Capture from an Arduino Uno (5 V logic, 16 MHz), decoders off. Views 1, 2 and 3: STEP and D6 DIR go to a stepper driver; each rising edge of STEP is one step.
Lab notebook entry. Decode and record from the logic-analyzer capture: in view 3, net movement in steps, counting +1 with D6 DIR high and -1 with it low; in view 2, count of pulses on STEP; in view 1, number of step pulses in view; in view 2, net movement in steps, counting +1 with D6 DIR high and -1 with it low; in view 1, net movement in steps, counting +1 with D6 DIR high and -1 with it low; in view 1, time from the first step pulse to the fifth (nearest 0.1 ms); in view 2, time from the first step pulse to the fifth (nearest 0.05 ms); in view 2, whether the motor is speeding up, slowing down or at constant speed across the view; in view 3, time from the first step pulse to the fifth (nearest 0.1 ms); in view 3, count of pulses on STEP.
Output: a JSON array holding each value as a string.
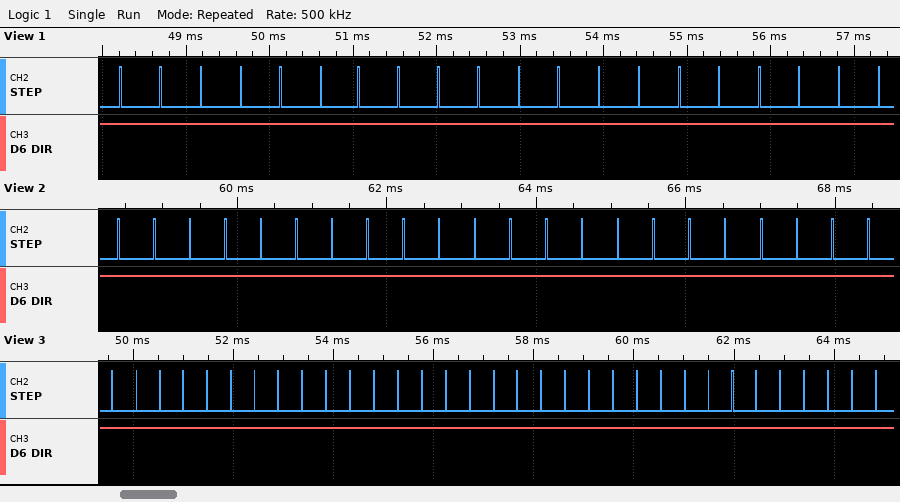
["+33", "22", "20", "+22", "+20", "1.9 ms", "1.90 ms", "constant speed", "1.9 ms", "33"]
